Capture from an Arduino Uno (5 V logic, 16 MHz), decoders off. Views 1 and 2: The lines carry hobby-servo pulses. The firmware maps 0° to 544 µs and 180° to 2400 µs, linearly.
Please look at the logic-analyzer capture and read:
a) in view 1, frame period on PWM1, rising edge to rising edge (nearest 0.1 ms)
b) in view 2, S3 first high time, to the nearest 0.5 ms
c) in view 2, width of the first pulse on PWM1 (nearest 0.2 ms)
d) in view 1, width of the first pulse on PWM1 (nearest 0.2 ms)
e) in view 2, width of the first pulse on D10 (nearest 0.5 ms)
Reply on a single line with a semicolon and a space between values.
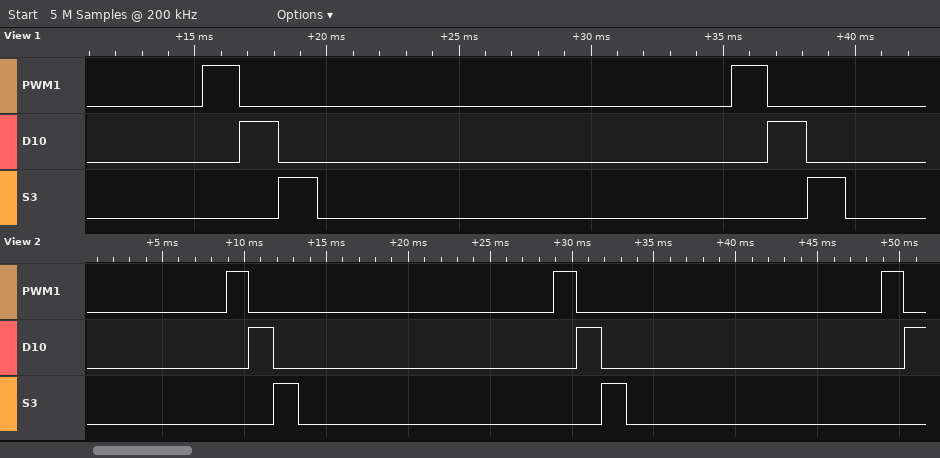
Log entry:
20.0 ms; 1.5 ms; 1.4 ms; 1.4 ms; 1.5 ms
